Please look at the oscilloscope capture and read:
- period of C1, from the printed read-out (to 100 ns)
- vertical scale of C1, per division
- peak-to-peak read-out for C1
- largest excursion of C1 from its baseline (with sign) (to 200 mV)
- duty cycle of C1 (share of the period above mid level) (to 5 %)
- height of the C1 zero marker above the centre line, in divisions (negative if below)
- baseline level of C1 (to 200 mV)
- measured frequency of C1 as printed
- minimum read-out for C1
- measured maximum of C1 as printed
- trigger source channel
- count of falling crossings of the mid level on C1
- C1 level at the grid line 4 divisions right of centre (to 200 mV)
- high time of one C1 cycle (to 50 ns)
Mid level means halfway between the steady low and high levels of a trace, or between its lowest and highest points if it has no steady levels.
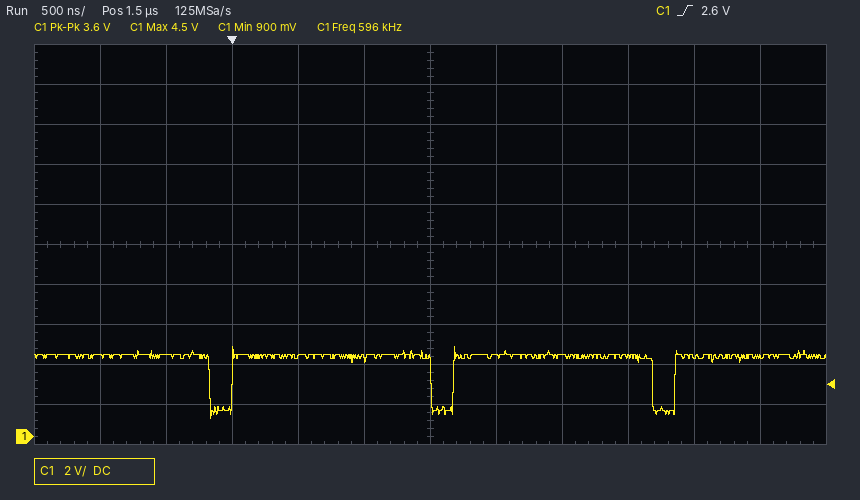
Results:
1.7 µs
2 V
3.6 V
-3.2 V
90 %
-4.8 div
4.0 V
596 kHz
900 mV
4.5 V
C1
3
4.0 V
1.50 µs
